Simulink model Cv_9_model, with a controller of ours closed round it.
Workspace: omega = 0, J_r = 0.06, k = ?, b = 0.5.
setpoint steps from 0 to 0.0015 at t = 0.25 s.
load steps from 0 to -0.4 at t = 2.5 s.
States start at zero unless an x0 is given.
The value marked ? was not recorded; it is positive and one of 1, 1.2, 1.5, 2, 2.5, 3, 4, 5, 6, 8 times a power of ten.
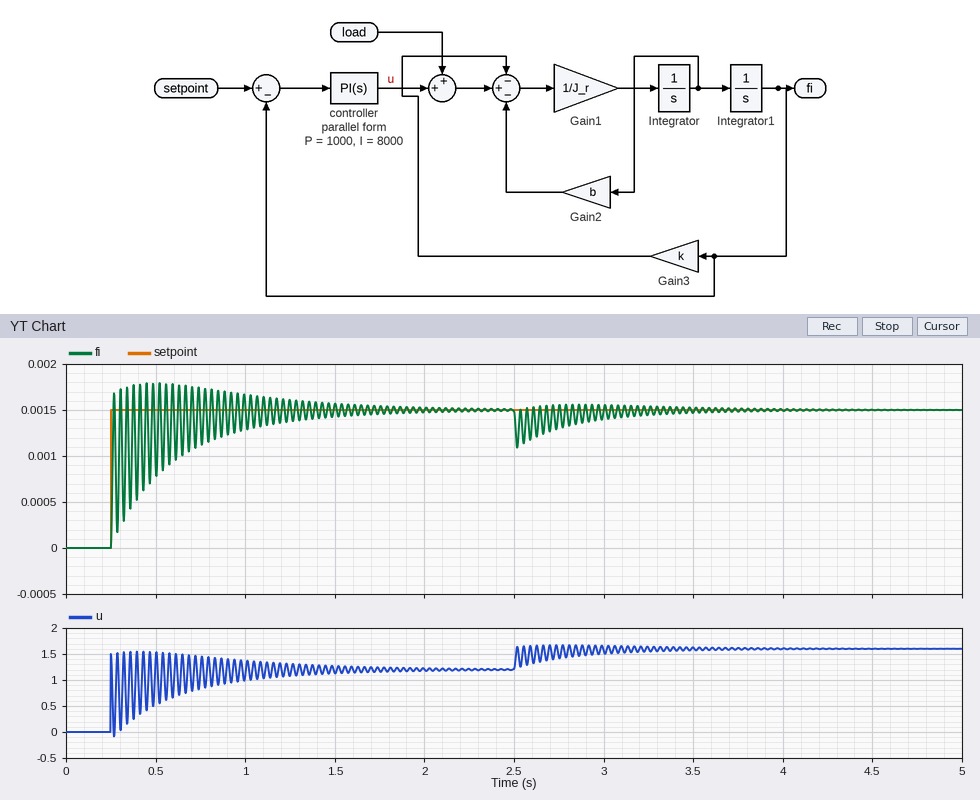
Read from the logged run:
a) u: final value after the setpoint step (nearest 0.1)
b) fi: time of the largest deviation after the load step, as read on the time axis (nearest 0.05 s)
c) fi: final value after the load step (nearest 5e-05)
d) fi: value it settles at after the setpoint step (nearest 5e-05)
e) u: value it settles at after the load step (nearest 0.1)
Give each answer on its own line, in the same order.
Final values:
1.2
2.50 s
0.00150
0.00150
1.6
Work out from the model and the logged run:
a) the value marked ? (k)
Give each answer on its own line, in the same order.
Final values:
800
